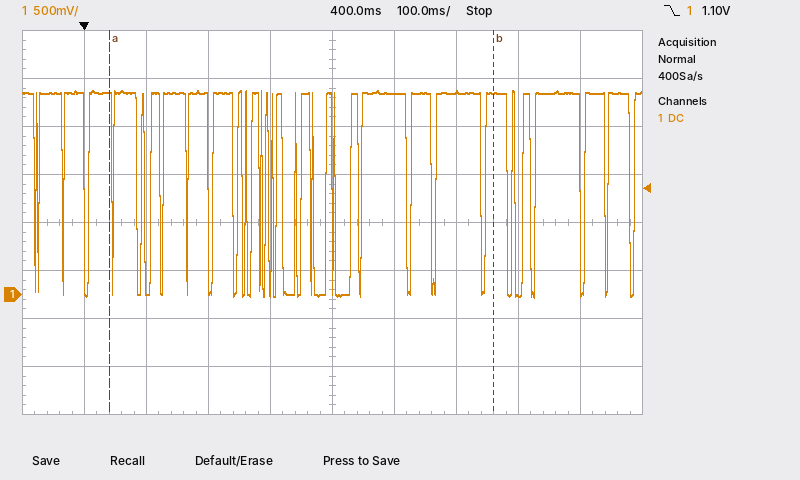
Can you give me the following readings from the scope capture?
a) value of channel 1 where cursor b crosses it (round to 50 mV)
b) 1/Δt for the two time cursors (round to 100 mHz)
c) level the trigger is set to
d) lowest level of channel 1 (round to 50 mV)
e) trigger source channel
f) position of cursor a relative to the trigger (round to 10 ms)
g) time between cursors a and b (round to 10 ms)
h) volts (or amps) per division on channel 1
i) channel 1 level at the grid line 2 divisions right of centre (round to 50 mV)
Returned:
2.10 V
1.6 Hz
1.10 V
-50 mV
channel 1
+40 ms
620 ms
500 mV
2.10 V
